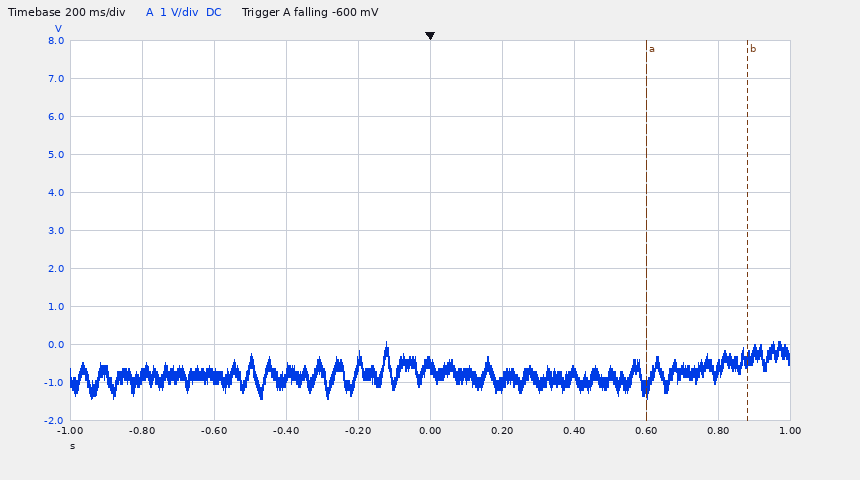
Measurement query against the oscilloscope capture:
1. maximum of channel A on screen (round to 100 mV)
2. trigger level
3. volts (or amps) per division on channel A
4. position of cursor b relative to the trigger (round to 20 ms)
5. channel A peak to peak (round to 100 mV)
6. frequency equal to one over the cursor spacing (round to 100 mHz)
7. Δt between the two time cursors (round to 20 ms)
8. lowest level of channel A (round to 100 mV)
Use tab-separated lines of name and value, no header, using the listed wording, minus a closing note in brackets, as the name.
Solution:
maximum of channel A on screen	100 mV
trigger level	-600 mV
volts (or amps) per division on channel A	1 V
position of cursor b relative to the trigger	+880 ms
channel A peak to peak	1.5 V
frequency equal to one over the cursor spacing	3.6 Hz
Δt between the two time cursors	280 ms
lowest level of channel A	-1.4 V
